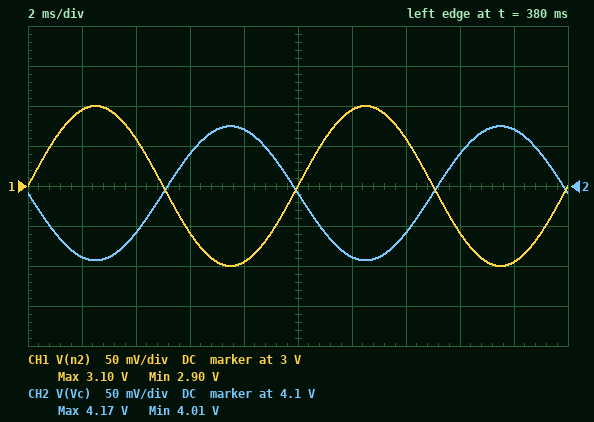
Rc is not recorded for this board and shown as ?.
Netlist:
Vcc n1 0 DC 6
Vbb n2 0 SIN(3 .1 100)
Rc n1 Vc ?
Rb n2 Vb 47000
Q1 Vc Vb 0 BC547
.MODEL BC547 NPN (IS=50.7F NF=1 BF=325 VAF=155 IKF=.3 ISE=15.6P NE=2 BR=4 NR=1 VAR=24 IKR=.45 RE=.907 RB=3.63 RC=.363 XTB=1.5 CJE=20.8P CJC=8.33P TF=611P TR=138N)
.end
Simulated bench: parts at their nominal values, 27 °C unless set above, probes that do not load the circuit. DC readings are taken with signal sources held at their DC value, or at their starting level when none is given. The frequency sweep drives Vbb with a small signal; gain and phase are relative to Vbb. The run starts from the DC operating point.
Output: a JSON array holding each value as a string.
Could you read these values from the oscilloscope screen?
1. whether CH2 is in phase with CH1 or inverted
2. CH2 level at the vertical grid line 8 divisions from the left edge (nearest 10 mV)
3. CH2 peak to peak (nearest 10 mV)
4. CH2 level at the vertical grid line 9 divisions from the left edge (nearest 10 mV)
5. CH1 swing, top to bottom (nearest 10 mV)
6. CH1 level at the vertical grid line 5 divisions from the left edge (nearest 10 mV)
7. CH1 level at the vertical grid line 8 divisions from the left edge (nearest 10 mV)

["inverted", "4.14 V", "170 mV", "4.17 V", "200 mV", "3.00 V", "2.94 V"]
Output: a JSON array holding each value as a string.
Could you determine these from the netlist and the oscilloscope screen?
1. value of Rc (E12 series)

["150 Ω"]
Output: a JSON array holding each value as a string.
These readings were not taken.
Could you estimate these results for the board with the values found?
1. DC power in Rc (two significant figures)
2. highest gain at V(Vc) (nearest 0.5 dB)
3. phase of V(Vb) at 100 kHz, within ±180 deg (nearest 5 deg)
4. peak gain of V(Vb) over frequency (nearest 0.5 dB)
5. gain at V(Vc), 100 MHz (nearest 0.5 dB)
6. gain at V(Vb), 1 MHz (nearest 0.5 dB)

["24 mW", "-1.5 dB", "-15 deg", "-35.5 dB", "-49.0 dB", "-43.5 dB"]
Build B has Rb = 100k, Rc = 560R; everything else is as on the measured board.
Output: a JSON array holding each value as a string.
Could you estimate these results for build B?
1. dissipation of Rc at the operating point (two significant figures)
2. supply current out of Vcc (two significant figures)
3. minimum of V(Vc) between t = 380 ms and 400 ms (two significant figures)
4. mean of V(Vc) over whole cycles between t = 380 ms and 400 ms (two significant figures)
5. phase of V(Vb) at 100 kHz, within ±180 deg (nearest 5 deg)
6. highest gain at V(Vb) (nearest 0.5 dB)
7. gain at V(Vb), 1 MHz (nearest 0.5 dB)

["18 mW", "5.7 mA", "2.7 V", "2.8 V", "-30 deg", "-36.5 dB", "-52.5 dB"]
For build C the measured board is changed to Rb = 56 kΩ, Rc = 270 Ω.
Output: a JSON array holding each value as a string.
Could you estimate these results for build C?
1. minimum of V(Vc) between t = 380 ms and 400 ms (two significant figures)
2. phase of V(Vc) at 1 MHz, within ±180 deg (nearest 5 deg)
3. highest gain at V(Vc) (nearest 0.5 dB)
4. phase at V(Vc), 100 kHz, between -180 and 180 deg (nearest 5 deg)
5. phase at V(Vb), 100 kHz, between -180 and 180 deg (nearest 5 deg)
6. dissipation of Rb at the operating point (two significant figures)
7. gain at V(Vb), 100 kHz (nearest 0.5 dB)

["3.0 V", "105 deg", "2.0 dB", "160 deg", "-20 deg", "96 µW", "-36.0 dB"]
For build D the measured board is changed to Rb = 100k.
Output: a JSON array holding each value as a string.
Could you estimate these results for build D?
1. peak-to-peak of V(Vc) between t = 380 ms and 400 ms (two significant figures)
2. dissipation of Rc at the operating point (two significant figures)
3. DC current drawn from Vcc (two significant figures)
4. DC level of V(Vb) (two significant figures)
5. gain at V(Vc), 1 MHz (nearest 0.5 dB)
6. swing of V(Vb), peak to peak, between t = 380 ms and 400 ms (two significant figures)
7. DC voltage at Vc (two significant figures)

["80 mV", "5.0 mW", "5.8 mA", "660 mV", "-16.5 dB", "3.0 mV", "5.1 V"]
